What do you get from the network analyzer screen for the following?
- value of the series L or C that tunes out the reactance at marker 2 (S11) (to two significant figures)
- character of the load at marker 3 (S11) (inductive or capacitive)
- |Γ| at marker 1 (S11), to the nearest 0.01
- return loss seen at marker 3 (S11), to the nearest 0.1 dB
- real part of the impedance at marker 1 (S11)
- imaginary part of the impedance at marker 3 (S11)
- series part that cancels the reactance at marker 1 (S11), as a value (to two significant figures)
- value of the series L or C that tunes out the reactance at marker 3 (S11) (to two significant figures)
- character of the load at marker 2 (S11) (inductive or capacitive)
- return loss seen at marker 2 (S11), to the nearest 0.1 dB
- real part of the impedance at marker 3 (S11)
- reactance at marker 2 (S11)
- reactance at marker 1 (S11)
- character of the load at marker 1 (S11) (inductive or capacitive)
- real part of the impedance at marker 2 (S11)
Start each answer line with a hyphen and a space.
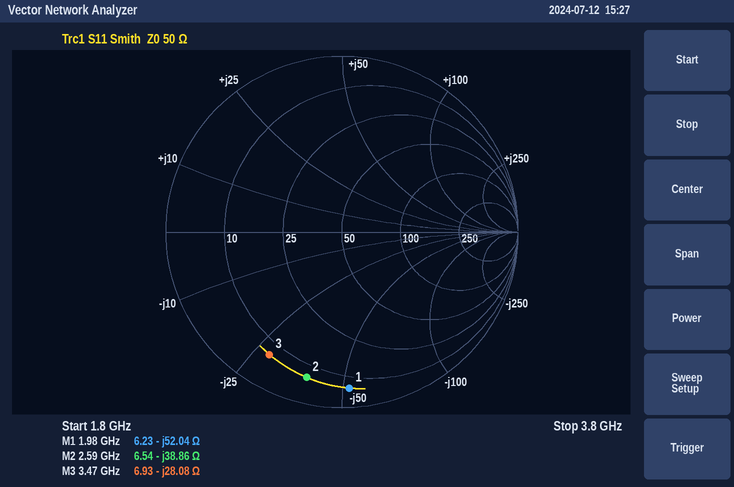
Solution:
- 2.4 nH
- capacitive
- 0.89
- 1.8 dB
- 6.23 Ω
- -28.08 Ω
- 4.2 nH
- 1.3 nH
- capacitive
- 1.4 dB
- 6.93 Ω
- -38.86 Ω
- -52.04 Ω
- capacitive
- 6.54 Ω
